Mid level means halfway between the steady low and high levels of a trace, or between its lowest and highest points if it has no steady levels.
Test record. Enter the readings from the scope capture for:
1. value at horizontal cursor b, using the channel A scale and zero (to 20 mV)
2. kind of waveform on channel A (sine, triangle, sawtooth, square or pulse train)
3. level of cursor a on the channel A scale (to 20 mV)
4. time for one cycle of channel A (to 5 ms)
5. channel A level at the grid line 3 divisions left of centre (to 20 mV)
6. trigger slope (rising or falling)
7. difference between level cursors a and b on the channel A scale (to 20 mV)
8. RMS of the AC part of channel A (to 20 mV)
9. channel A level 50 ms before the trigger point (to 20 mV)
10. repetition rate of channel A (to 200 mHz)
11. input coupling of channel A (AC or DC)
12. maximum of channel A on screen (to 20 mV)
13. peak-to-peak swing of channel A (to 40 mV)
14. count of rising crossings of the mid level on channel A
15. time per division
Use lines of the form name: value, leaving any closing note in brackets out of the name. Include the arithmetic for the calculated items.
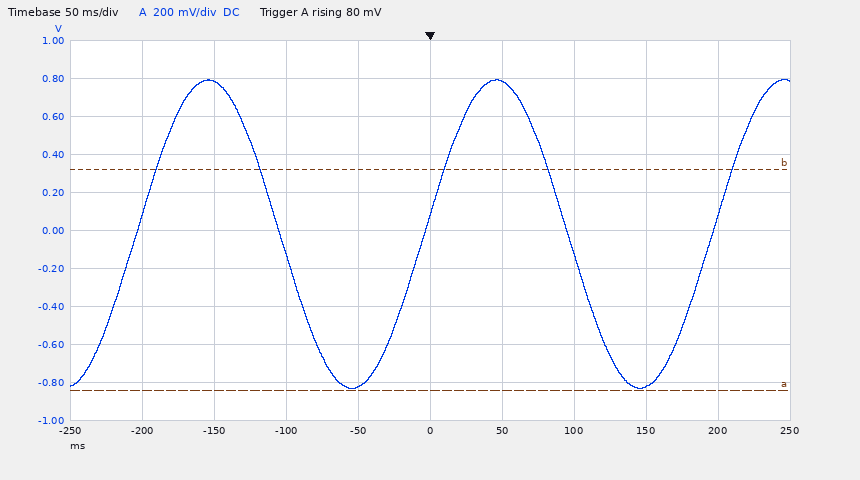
value at horizontal cursor b, using the channel A scale and zero: 320 mV
kind of waveform on channel A: sine
level of cursor a on the channel A scale: -840 mV
time for one cycle of channel A: 200 ms
channel A level at the grid line 3 divisions left of centre: 780 mV
trigger slope: rising
difference between level cursors a and b on the channel A scale: 1.16 V
RMS of the AC part of channel A: 1.64 V / (2√2) ≈ 580 mV
channel A level 50 ms before the trigger point: -820 mV
repetition rate of channel A: 1 / 200 ms ≈ 5.0 Hz
input coupling of channel A: DC
maximum of channel A on screen: 800 mV
peak-to-peak swing of channel A: 1.64 V
count of rising crossings of the mid level on channel A: 3
time per division: 50 ms
